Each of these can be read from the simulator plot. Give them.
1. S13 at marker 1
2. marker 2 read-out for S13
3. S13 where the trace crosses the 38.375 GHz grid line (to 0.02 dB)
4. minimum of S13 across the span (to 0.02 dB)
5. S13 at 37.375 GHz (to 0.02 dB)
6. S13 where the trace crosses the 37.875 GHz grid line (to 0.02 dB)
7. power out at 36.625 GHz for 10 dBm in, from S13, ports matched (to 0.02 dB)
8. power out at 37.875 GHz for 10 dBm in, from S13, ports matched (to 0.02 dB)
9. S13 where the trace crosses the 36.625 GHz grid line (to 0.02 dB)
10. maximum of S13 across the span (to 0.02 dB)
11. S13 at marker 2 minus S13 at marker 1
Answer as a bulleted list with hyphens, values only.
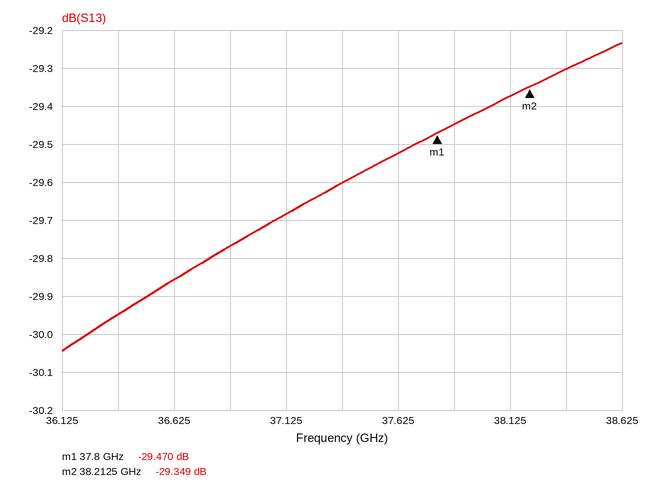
- -29.470 dB
- -29.349 dB
- -29.30 dB
- -30.04 dB
- -29.60 dB
- -29.44 dB
- -19.86 dBm
- -19.44 dBm
- -29.86 dB
- -29.24 dB
- 0.121 dB
